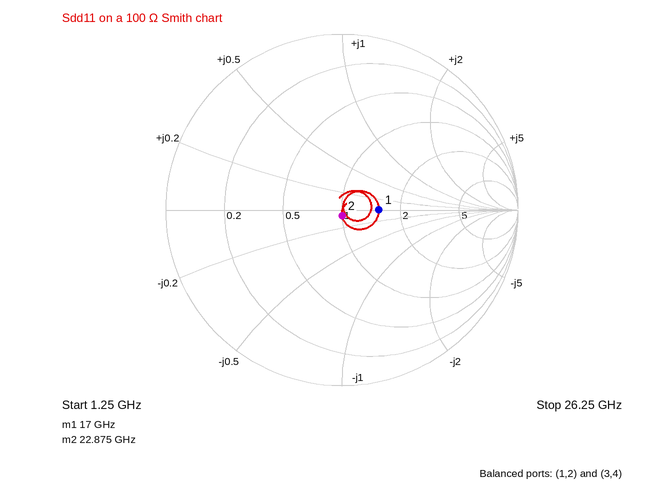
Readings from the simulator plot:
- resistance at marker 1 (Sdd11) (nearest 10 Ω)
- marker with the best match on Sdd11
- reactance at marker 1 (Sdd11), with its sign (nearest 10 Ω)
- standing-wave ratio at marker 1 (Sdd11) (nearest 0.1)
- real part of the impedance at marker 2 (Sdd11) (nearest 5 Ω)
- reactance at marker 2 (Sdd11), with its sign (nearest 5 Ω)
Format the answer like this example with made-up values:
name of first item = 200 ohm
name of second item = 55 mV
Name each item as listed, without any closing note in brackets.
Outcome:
resistance at marker 1 (Sdd11) = 150 Ω
marker with the best match on Sdd11 = marker 2
reactance at marker 1 (Sdd11), with its sign = 0 Ω
standing-wave ratio at marker 1 (Sdd11) = 1.5
real part of the impedance at marker 2 (Sdd11) = 100 Ω
reactance at marker 2 (Sdd11), with its sign = -5 Ω
